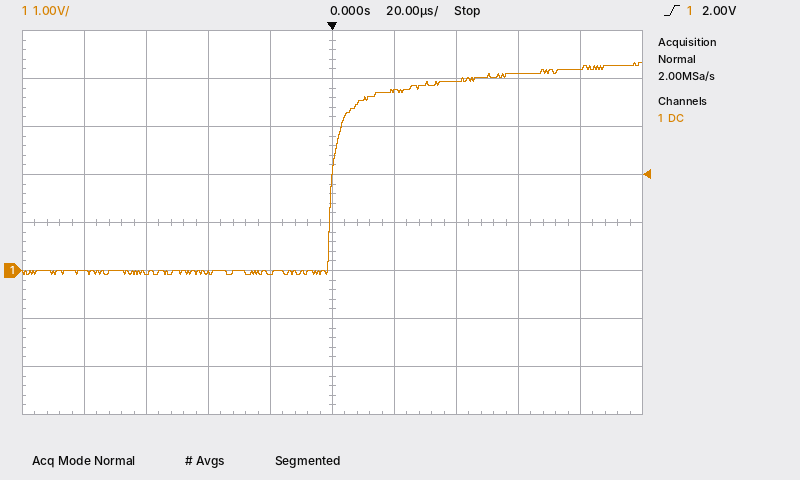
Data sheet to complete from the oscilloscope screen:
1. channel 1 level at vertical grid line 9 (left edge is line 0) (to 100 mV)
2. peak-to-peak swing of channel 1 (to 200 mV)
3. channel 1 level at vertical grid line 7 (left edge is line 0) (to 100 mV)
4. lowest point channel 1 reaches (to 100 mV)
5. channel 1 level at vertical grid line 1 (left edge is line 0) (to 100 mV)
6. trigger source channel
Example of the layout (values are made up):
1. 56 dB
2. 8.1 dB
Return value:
1. 4.2 V
2. 4.4 V
3. 3.9 V
4. -100 mV
5. 0.0 V
6. channel 1
